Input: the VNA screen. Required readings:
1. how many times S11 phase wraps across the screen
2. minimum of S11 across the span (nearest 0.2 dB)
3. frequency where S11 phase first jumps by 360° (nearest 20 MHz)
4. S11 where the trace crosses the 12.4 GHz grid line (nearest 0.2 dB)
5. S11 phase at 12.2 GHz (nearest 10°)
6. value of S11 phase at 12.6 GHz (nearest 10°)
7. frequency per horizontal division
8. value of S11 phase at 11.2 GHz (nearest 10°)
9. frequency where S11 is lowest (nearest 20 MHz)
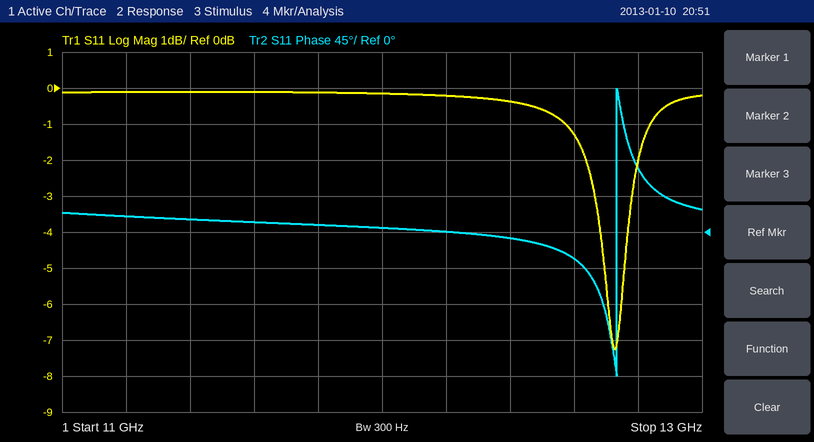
1
-7.2 dB
12.74 GHz
-0.4 dB
0°
-30°
200 MHz
20°
12.72 GHz
